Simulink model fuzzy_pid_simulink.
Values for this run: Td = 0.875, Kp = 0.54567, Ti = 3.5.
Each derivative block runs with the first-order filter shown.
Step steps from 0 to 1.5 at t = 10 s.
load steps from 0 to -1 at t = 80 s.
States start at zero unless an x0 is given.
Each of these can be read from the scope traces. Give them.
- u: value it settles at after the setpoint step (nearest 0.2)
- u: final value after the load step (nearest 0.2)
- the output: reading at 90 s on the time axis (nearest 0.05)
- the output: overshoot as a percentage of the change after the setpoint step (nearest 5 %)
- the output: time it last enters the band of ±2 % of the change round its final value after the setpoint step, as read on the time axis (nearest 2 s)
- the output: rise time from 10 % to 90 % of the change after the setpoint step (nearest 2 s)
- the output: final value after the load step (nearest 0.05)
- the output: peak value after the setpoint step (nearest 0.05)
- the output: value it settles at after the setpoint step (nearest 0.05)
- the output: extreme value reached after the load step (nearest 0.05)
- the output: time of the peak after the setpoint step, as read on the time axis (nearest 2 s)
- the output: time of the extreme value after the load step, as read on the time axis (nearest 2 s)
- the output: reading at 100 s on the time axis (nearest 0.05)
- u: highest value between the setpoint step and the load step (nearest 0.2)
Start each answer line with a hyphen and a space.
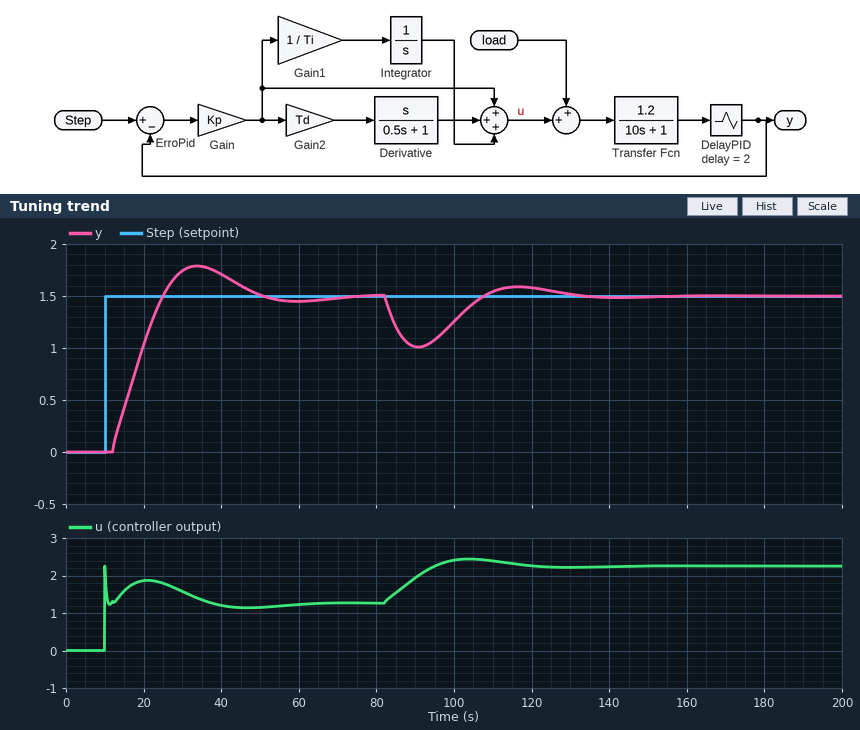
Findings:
- 1.2
- 2.2
- 1.00
- 20 %
- 68 s
- 10 s
- 1.50
- 1.80
- 1.50
- 1.00
- 34 s
- 90 s
- 1.25
- 2.2
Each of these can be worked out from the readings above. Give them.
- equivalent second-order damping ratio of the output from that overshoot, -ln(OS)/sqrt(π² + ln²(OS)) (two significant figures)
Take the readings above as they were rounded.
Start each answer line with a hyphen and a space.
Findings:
- 0.46
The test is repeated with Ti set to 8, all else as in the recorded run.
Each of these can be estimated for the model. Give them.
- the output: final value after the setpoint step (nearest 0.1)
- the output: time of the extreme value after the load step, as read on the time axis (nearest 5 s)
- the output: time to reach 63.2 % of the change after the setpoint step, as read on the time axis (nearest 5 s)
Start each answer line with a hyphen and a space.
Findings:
- 1.5
- 95 s
- 25 s
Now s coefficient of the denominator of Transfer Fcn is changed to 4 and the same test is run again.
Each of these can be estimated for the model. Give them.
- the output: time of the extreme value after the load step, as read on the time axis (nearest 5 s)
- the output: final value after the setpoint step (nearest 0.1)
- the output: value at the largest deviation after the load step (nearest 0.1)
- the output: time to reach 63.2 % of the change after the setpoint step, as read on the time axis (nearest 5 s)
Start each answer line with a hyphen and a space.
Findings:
- 85 s
- 1.5
- 0.9
- 15 s
